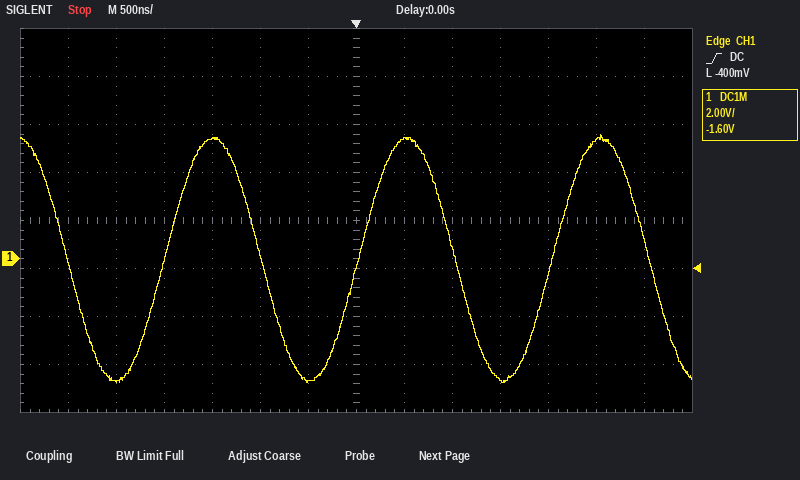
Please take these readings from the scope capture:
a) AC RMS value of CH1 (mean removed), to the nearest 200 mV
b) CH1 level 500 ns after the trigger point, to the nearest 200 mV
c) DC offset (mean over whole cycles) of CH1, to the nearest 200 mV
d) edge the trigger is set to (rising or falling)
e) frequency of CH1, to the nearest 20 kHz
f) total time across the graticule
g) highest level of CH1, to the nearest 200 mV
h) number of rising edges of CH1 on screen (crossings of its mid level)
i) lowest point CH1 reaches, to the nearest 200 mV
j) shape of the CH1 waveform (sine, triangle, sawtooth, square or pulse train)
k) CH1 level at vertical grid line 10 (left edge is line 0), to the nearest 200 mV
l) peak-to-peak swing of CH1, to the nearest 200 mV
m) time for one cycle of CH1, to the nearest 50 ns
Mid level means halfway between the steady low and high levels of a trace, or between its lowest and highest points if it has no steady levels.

3.6 V
5.0 V
0.0 V
rising
500 kHz
7 µs
5.2 V
3
-5.2 V
sine
-5.0 V
10.4 V
2.00 µs
